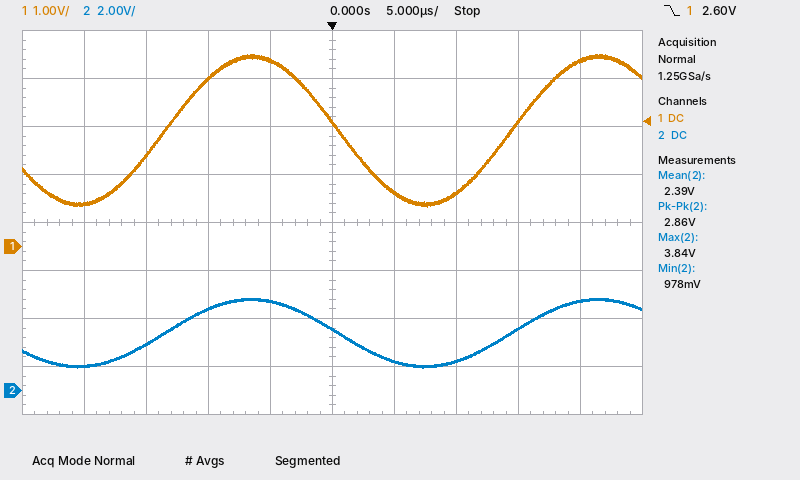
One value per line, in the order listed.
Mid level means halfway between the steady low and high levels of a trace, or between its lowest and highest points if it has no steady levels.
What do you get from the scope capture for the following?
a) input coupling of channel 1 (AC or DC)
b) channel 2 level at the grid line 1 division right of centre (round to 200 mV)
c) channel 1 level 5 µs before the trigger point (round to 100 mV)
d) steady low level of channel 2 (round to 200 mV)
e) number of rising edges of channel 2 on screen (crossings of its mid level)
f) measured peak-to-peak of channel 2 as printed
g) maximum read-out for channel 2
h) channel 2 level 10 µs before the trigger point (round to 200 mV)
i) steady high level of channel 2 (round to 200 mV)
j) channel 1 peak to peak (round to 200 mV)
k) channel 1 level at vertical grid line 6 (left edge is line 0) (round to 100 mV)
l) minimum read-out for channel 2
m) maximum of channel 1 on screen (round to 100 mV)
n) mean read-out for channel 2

DC
1.2 V
3.9 V
1.0 V
2
2.86 V
3.84 V
3.4 V
3.8 V
3.2 V
1.1 V
978 mV
4.0 V
2.39 V
